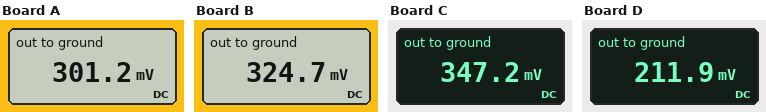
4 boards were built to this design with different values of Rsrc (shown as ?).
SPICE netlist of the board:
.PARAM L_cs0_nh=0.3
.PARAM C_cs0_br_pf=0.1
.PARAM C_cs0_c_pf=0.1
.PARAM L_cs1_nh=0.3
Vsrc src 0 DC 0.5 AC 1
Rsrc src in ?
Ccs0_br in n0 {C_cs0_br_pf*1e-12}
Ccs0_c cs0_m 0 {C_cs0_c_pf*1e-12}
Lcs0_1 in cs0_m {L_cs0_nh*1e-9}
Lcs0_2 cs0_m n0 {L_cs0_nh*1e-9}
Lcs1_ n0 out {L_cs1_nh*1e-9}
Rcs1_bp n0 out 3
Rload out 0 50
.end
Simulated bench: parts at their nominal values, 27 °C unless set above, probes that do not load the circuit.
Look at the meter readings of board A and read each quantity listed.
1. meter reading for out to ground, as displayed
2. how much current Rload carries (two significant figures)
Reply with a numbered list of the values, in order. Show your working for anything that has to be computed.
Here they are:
1. 301.2 mV
2. (301.2 mV) / 50 Ω = 6.0 mA
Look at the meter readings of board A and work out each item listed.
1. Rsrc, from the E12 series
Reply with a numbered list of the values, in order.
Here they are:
1. 33 Ω
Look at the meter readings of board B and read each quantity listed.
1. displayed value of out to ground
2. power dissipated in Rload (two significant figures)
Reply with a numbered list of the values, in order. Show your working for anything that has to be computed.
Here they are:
1. 324.7 mV
2. (324.7 mV)^2 / 50 Ω = 2.1 mW
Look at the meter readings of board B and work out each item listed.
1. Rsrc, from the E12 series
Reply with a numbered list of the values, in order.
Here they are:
1. 27 Ω
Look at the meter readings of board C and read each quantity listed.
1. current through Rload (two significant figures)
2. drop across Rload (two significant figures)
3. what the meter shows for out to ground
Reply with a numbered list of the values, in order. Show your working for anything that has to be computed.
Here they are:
1. (347.2 mV) / 50 Ω = 6.9 mA
2. 347.2 mV = 350 mV
3. 347.2 mV
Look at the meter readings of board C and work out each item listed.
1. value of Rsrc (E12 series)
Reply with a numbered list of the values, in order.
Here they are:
1. 22 Ω
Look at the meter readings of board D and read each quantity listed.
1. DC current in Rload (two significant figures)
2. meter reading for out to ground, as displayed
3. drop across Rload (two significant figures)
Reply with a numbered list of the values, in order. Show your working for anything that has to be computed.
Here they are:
1. (211.9 mV) / 50 Ω = 4.2 mA
2. 211.9 mV
3. 211.9 mV = 210 mV
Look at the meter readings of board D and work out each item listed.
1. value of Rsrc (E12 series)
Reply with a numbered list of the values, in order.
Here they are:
1. 68 Ω
